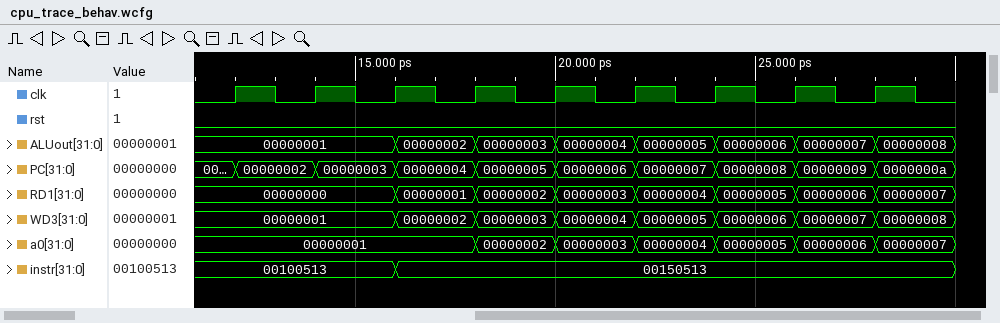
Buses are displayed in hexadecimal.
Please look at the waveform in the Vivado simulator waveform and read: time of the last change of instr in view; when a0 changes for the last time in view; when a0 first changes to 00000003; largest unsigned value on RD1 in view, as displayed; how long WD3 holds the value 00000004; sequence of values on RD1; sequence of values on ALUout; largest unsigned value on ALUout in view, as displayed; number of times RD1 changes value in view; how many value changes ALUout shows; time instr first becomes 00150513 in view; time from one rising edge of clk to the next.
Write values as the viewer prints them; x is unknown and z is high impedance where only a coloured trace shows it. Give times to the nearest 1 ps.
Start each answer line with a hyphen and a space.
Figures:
- 16 ps
- 28 ps
- 20 ps
- 00000007
- 2 ps
- 00000000, 00000001, 00000002, 00000003, 00000004, 00000005, 00000006, 00000007
- 00000001, 00000002, 00000003, 00000004, 00000005, 00000006, 00000007, 00000008
- 00000008
- 7
- 7
- 16 ps
- 2 ps
